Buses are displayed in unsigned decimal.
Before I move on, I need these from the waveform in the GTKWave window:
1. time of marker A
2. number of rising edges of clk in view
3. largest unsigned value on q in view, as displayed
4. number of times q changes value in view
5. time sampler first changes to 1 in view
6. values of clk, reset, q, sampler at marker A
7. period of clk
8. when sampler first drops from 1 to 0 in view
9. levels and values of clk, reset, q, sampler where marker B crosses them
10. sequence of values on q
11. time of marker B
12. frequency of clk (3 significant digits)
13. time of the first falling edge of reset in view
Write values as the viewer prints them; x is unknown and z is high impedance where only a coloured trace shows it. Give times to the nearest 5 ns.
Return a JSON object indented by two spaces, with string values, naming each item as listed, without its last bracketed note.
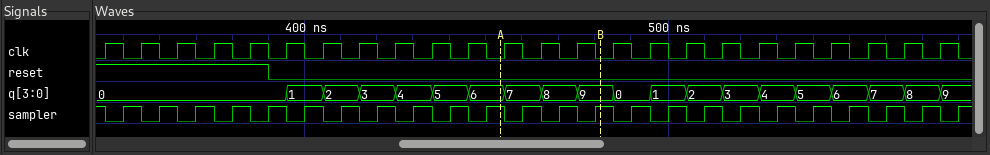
{
  "time of marker A": "455 ns",
  "number of rising edges of clk in view": "24",
  "largest unsigned value on q in view, as displayed": "9",
  "number of times q changes value in view": "19",
  "time sampler first changes to 1 in view": "350 ns",
  "values of clk, reset, q, sampler at marker A": "clk=0, reset=0, q=6, sampler=1",
  "period of clk": "10 ns",
  "when sampler first drops from 1 to 0 in view": "345 ns",
  "levels and values of clk, reset, q, sampler where marker B crosses them": "clk=0, reset=0, q=9, sampler=1",
  "sequence of values on q": "0, 1, 2, 3, 4, 5, 6, 7, 8, 9, 0, 1, 2, 3, 4, 5, 6, 7, 8, 9",
  "time of marker B": "480 ns",
  "frequency of clk": "100 MHz",
  "time of the first falling edge of reset in view": "390 ns"
}
